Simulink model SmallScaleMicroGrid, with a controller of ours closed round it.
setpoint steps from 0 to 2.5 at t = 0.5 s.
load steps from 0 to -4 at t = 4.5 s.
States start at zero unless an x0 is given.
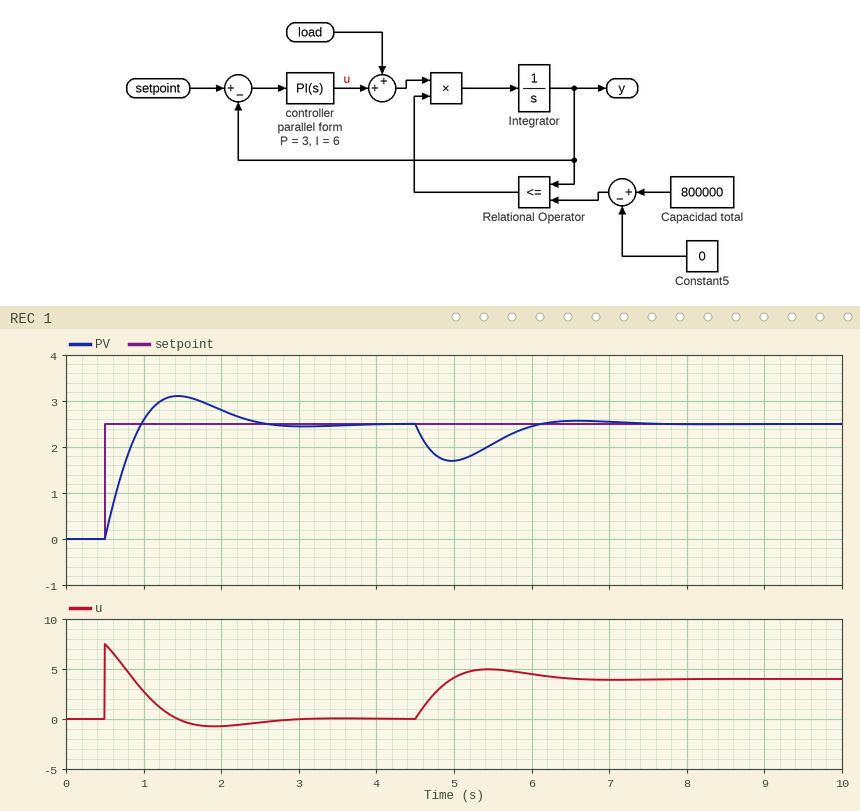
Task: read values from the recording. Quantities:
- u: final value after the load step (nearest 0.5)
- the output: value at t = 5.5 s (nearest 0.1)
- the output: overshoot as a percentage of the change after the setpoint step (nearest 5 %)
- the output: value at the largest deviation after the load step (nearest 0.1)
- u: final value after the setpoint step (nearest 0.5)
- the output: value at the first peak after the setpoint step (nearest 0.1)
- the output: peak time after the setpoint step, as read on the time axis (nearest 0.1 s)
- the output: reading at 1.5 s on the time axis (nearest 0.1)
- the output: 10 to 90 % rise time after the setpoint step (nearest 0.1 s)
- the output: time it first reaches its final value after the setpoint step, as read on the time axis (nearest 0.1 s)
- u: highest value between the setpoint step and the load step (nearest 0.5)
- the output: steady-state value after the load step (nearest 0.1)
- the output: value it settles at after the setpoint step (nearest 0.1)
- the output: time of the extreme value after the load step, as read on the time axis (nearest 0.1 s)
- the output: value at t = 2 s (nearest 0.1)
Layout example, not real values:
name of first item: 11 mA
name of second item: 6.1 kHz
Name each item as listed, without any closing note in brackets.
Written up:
u: final value after the load step: 4.0
the output: value at t = 5.5 s: 2.1
the output: overshoot as a percentage of the change after the setpoint step: 25 %
the output: value at the largest deviation after the load step: 1.7
u: final value after the setpoint step: 0.0
the output: value at the first peak after the setpoint step: 3.1
the output: peak time after the setpoint step, as read on the time axis: 1.4 s
the output: reading at 1.5 s on the time axis: 3.1
the output: 10 to 90 % rise time after the setpoint step: 0.4 s
the output: time it first reaches its final value after the setpoint step, as read on the time axis: 1.0 s
u: highest value between the setpoint step and the load step: 7.5
the output: steady-state value after the load step: 2.5
the output: value it settles at after the setpoint step: 2.5
the output: time of the extreme value after the load step, as read on the time axis: 5.0 s
the output: value at t = 2 s: 2.8
